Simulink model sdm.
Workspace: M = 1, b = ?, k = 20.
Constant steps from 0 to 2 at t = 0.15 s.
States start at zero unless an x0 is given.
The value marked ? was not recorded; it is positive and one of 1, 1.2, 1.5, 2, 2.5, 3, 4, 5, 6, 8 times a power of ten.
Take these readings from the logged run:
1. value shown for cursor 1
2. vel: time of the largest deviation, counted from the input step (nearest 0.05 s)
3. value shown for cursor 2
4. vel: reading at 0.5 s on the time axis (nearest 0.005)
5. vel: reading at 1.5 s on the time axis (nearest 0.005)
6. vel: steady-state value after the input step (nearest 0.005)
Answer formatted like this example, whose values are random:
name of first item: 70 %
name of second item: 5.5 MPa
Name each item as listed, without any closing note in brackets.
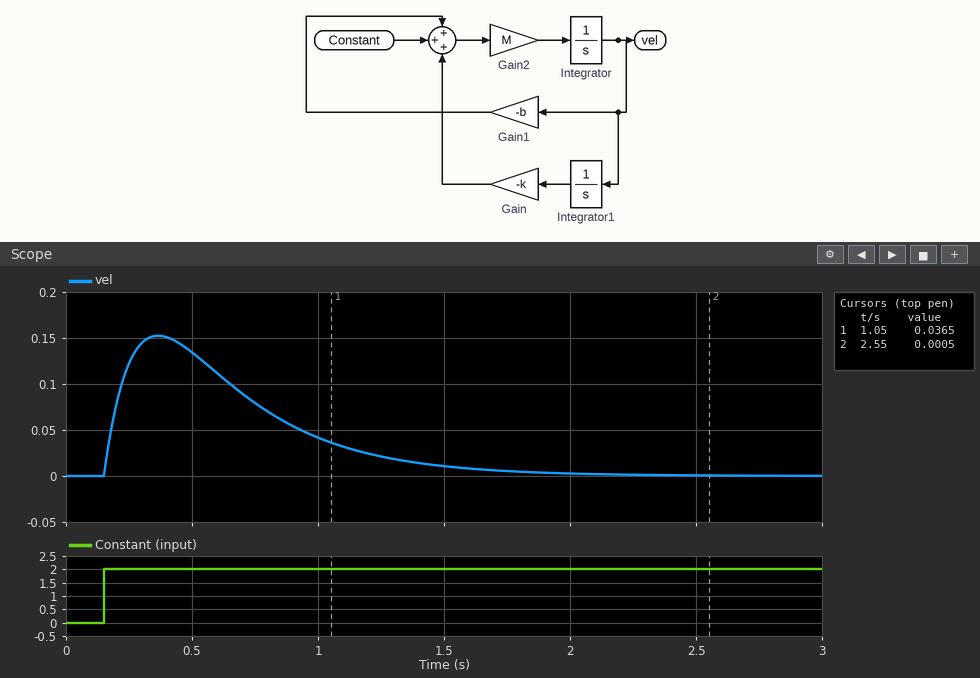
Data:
value shown for cursor 1: 0.0365
vel: time of the largest deviation, counted from the input step: 0.20 s
value shown for cursor 2: 0.0005
vel: reading at 0.5 s on the time axis: 0.135
vel: reading at 1.5 s on the time axis: 0.010
vel: steady-state value after the input step: 0.000
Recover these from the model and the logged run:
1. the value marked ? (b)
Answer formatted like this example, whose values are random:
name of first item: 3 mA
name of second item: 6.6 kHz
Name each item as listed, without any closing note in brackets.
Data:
the value marked ?: 10
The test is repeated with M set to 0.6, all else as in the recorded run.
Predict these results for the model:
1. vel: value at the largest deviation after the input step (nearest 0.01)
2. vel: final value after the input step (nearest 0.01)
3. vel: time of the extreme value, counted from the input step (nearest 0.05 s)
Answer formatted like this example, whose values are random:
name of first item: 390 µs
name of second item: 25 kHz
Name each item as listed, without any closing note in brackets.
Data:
vel: value at the largest deviation after the input step: 0.14
vel: final value after the input step: 0.00
vel: time of the extreme value, counted from the input step: 0.30 s
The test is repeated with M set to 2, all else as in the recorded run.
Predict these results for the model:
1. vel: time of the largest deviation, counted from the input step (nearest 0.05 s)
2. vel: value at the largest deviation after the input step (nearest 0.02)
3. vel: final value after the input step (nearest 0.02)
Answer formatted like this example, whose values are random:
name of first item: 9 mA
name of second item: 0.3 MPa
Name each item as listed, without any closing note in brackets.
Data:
vel: time of the largest deviation, counted from the input step: 0.15 s
vel: value at the largest deviation after the input step: 0.16
vel: final value after the input step: 0.00
